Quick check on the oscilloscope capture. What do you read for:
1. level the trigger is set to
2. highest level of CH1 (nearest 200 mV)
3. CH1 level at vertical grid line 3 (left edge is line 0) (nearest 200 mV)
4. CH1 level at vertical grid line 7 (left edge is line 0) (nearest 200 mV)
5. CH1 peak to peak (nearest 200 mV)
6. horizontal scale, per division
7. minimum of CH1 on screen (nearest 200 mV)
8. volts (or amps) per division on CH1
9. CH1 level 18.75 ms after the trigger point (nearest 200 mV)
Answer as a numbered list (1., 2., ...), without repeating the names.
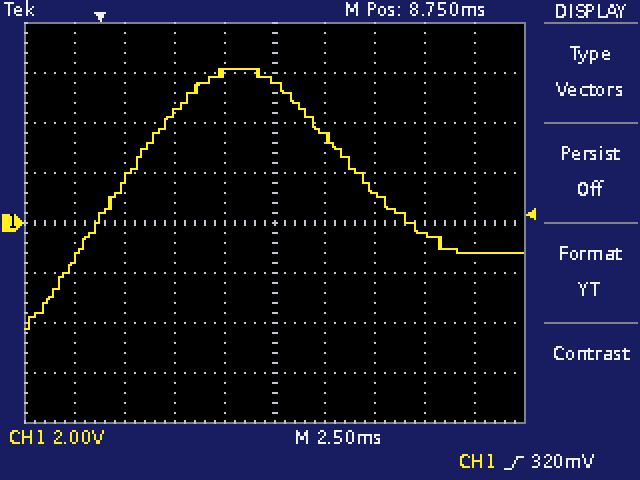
1. 320 mV
2. 6.2 V
3. 4.4 V
4. 1.2 V
5. 10.4 V
6. 2.5 ms
7. -4.2 V
8. 2 V
9. -1.2 V
